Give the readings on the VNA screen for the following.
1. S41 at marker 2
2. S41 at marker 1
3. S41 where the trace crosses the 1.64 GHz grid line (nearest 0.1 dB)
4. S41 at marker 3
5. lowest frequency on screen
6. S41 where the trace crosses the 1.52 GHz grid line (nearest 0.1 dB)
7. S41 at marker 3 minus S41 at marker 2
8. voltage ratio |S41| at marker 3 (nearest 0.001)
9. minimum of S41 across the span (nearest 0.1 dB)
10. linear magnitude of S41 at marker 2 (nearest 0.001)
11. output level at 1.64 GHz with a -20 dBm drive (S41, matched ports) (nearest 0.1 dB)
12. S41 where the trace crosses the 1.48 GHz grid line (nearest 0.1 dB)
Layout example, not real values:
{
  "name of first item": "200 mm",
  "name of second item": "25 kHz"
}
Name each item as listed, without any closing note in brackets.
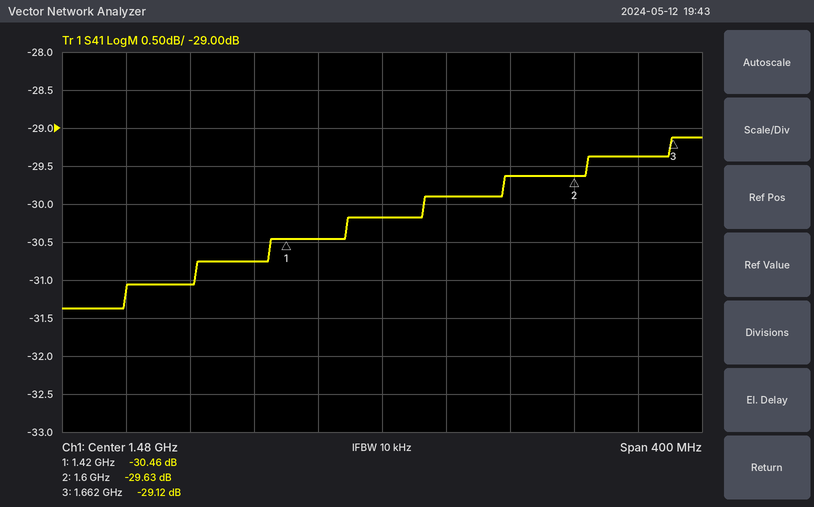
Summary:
{
  "S41 at marker 2": "-29.63 dB",
  "S41 at marker 1": "-30.46 dB",
  "S41 where the trace crosses the 1.64 GHz grid line": "-29.4 dB",
  "S41 at marker 3": "-29.12 dB",
  "lowest frequency on screen": "1.28 GHz",
  "S41 where the trace crosses the 1.52 GHz grid line": "-29.9 dB",
  "S41 at marker 3 minus S41 at marker 2": "0.51 dB",
  "voltage ratio |S41| at marker 3": "0.035",
  "minimum of S41 across the span": "-31.4 dB",
  "linear magnitude of S41 at marker 2": "0.033",
  "output level at 1.64 GHz with a -20 dBm drive (S41, matched ports)": "-49.4 dBm",
  "S41 where the trace crosses the 1.48 GHz grid line": "-30.2 dB"
}
